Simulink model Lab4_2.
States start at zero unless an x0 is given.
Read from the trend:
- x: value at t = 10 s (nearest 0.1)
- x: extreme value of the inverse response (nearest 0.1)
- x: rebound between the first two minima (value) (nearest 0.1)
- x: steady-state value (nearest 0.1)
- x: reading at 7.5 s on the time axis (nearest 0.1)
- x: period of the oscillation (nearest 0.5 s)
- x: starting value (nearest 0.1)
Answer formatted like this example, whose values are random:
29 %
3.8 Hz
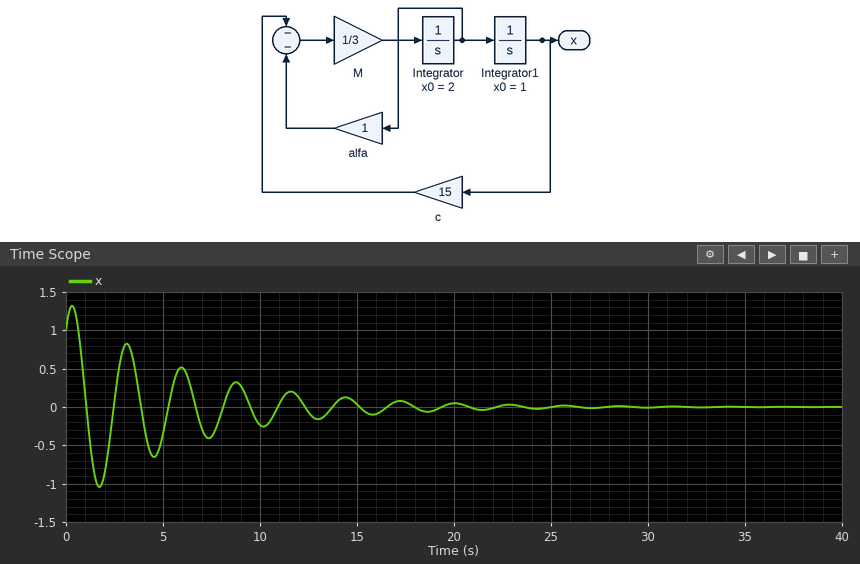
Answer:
-0.2
1.3
0.8
0.0
-0.4
3.0 s
1.0
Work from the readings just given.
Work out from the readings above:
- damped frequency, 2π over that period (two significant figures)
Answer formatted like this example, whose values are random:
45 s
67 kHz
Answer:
2.1 rad/s
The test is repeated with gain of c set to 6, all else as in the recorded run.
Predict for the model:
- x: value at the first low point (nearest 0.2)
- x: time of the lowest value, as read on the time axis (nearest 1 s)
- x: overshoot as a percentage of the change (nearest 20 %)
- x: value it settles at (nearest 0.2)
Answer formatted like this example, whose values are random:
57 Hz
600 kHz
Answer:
-1.2
3 s
120 %
0.0
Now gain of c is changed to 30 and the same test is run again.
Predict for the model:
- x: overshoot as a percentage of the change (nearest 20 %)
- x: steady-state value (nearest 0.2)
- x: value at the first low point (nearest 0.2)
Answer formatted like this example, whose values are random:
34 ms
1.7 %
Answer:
100 %
0.0
-1.0
